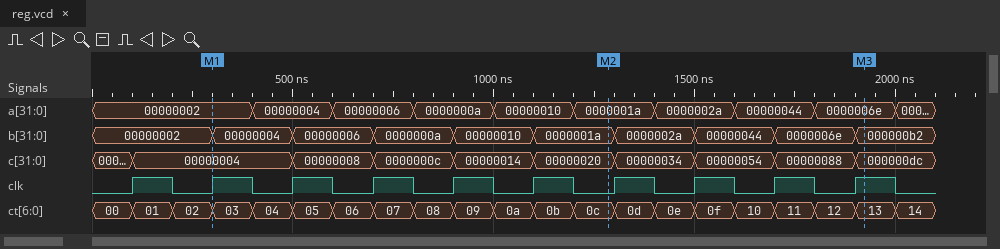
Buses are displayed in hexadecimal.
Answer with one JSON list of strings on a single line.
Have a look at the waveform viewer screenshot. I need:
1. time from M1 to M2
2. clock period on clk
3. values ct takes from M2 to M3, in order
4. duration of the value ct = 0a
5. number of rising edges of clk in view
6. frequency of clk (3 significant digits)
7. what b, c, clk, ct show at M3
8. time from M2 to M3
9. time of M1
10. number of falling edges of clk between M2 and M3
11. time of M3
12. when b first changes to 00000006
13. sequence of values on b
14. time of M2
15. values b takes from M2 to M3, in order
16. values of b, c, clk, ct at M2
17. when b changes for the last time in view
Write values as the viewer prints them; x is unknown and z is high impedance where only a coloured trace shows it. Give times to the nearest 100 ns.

["1000 ns", "200 ns", "0c, 0d, 0e, 0f, 10, 11, 12, 13", "100 ns", "10", "5.00 MHz", "b=000000b2, c=000000dc, clk=1, ct=13", "600 ns", "300 ns", "3", "1900 ns", "500 ns", "00000002, 00000004, 00000006, 0000000a, 00000010, 0000001a, 0000002a, 00000044, 0000006e, 000000b2", "1300 ns", "0000001a, 0000002a, 00000044, 0000006e, 000000b2", "b=0000001a, c=00000020, clk=0, ct=0c", "1900 ns"]
